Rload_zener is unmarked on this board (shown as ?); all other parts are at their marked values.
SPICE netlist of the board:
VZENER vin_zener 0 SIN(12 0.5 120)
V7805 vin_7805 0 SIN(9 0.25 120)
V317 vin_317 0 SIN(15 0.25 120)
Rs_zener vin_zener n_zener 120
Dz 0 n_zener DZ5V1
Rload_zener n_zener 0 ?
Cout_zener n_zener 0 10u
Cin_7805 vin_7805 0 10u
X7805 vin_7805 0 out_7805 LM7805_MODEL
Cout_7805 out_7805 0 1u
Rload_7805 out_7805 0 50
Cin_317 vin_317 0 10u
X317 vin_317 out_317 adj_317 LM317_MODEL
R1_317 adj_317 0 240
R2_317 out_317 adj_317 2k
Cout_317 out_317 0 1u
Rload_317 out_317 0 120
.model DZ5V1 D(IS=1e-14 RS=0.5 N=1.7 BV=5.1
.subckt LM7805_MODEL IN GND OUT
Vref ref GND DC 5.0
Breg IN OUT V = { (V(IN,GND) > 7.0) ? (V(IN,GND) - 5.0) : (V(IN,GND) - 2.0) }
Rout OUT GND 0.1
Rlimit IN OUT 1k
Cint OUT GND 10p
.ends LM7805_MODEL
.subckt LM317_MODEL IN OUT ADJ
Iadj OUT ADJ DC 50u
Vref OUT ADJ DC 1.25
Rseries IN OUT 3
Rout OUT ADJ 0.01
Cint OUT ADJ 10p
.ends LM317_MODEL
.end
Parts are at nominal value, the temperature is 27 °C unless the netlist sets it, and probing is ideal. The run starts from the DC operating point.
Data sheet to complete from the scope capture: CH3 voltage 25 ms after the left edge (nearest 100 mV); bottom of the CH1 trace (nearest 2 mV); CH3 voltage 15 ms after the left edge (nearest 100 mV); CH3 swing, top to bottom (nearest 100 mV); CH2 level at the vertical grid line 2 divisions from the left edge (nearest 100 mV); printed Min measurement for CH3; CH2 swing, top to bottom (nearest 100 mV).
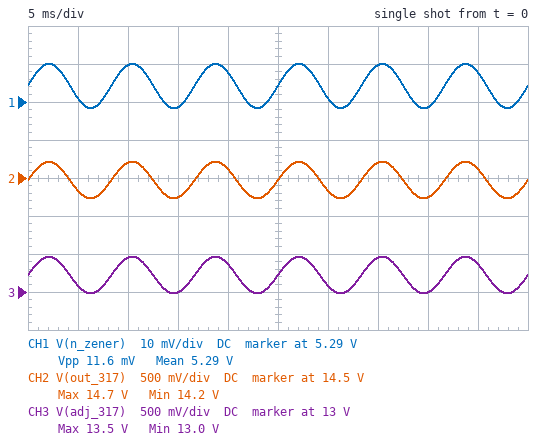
13.2 V
5.288 V
13.0 V
500 mV
14.7 V
13.0 V
500 mV
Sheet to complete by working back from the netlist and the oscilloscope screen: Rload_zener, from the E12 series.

680 Ω
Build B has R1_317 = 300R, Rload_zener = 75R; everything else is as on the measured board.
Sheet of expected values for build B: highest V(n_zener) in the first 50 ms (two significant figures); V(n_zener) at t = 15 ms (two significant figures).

4.8 V
4.4 V
